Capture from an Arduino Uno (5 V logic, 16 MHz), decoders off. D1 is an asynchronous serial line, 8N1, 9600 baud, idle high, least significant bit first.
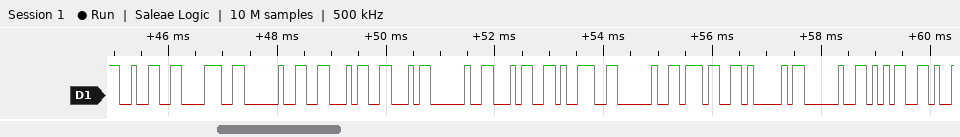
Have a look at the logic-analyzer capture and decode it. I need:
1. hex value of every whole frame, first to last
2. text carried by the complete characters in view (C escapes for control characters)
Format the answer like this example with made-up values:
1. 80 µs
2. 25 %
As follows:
1. 32 38 20 46 46 20 34 39 20 37 41 20 35
2. "28 FF 49 7A 5"
